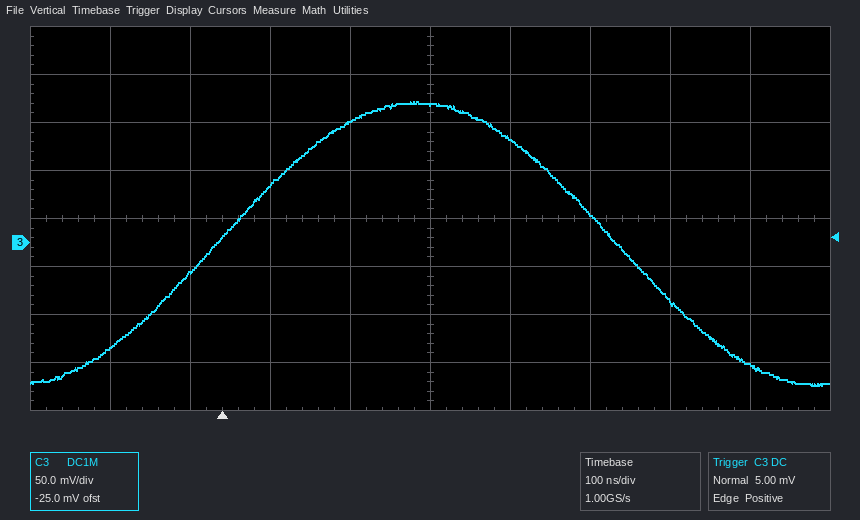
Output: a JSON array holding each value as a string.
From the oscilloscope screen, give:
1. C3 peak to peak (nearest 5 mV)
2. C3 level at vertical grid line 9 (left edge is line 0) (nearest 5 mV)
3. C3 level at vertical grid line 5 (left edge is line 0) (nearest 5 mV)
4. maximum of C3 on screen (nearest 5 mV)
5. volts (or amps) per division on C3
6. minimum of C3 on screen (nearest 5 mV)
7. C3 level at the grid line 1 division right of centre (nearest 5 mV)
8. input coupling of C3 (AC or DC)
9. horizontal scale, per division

["295 mV", "-130 mV", "145 mV", "145 mV", "50 mV", "-150 mV", "110 mV", "DC", "100 ns"]
